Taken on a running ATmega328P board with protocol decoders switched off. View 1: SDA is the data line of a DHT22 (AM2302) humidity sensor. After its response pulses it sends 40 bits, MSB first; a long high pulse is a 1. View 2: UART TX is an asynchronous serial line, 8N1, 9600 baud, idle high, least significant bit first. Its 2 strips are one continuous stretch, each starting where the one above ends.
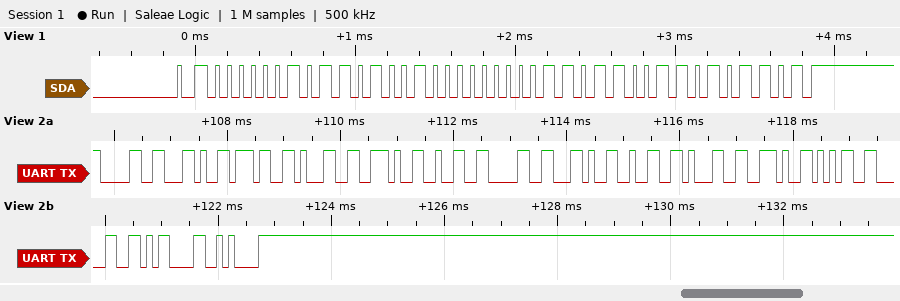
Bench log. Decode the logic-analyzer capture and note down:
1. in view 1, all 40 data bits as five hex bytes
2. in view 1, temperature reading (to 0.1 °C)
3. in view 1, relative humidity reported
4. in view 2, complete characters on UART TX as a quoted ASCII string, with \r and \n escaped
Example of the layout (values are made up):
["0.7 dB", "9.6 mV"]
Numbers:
["02 D2 00 D9 AD", "21.7 °C", "72.2 %", "\"0,71.20,21.50\\r\\n\""]
